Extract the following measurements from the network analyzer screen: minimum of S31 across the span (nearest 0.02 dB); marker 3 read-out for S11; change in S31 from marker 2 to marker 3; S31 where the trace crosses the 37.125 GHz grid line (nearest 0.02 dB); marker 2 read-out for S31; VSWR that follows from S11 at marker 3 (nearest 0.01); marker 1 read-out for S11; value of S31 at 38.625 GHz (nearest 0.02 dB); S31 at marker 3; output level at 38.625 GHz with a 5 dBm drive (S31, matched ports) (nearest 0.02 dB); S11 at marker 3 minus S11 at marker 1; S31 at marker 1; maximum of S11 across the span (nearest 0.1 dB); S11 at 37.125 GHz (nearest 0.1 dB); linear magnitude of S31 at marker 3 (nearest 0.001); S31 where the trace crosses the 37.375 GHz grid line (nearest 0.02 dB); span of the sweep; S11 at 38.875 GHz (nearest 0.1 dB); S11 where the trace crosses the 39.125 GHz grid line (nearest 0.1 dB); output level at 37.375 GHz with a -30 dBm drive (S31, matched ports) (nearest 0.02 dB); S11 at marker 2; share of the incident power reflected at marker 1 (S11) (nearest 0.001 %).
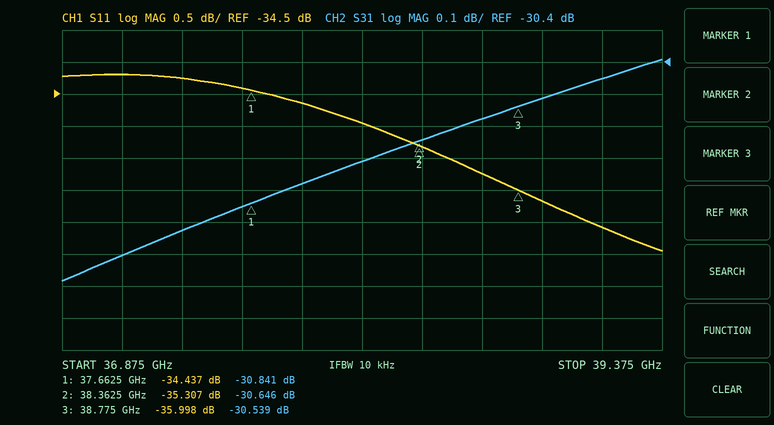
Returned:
-31.08 dB
-35.998 dB
0.107 dB
-31.00 dB
-30.646 dB
1.03
-34.437 dB
-30.58 dB
-30.539 dB
-25.58 dBm
-1.561 dB
-30.841 dB
-34.2 dB
-34.2 dB
0.030
-30.92 dB
2.5 GHz
-36.2 dB
-36.6 dB
-60.92 dBm
-35.307 dB
0.036 %
